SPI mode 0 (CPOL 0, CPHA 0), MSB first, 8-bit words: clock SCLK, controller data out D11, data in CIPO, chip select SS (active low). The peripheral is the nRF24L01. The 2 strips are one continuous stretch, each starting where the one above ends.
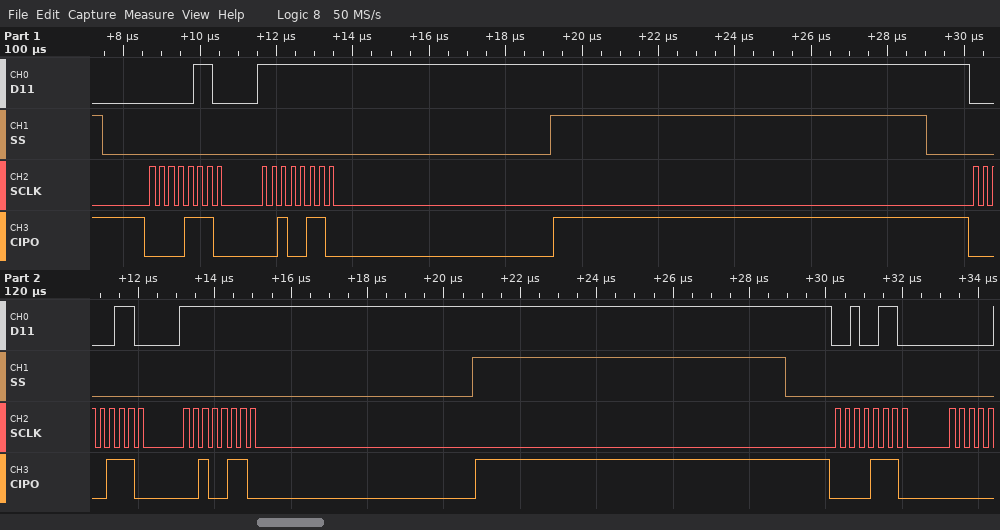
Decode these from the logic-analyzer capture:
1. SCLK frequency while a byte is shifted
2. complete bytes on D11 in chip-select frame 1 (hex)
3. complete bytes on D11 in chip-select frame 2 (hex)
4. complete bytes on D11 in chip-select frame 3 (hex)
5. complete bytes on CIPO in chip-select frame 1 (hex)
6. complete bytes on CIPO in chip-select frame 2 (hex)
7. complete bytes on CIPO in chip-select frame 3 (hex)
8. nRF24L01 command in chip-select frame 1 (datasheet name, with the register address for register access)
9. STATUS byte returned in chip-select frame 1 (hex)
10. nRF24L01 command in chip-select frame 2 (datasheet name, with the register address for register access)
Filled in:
4 MHz
0x06 0xFF
0x06 0xFF
0x26
0x0E 0x26
0x0E 0x26
0x0E
R_REGISTER 0x06
0x0E
R_REGISTER 0x06
